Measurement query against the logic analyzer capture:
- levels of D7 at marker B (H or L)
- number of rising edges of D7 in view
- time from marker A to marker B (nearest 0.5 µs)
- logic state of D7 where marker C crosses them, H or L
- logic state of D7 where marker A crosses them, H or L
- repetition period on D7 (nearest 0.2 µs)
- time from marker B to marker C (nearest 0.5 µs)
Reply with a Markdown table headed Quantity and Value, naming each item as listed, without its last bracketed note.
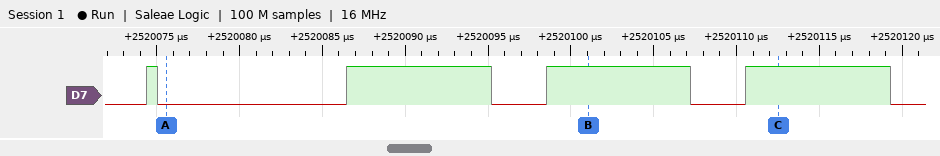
| Quantity | Value |
|---|---|
| levels of D7 at marker B | D7=H |
| number of rising edges of D7 in view | 4 |
| time from marker A to marker B | 25.5 µs |
| logic state of D7 where marker C crosses them, H or L | D7=H |
| logic state of D7 where marker A crosses them, H or L | D7=L |
| repetition period on D7 | 12 µs |
| time from marker B to marker C | 11.5 µs |
